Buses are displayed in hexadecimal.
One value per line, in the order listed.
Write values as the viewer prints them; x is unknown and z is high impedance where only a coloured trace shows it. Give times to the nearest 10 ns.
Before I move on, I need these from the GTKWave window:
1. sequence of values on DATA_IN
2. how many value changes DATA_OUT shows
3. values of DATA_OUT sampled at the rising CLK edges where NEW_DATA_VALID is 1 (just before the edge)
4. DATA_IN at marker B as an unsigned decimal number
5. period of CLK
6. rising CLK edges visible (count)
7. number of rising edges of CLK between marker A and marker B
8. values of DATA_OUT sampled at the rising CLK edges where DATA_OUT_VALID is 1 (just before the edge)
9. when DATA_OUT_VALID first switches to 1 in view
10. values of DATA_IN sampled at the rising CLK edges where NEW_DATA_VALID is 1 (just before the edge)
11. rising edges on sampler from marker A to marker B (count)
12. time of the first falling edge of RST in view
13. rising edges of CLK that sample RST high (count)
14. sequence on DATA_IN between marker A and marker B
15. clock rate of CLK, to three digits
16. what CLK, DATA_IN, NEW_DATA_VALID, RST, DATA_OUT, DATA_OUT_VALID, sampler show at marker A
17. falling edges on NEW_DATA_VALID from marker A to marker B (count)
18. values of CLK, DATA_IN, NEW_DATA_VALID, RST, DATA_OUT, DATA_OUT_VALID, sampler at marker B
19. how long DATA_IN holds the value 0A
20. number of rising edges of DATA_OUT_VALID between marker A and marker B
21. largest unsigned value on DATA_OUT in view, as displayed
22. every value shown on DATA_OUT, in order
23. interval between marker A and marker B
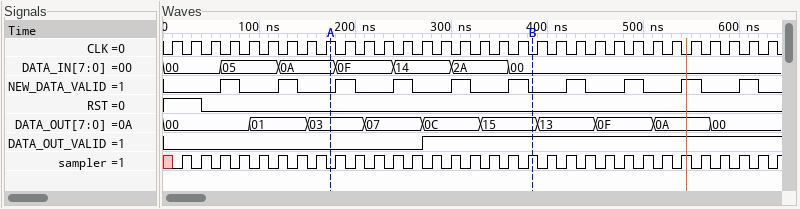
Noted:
00, 05, 0A, 0F, 14, 2A, 00
9
00, 01, 03, 07, 0C, 15, 13, 0F, 0A, 00
0
20 ns
32
10
0C, 0C, 0C, 15, 15, 15, 13, 13, 13, 0F, 0F, 0F, 0A, 0A, 0A, 00, 00, 00
270 ns
05, 0A, 0F, 14, 2A, 00, 00, 00, 00, 00
11
40 ns
2
0A, 0F, 14, 2A, 00
50.0 MHz
CLK=1, DATA_IN=0A, NEW_DATA_VALID=0, RST=0, DATA_OUT=03, DATA_OUT_VALID=0, sampler=0
4
CLK=0, DATA_IN=00, NEW_DATA_VALID=0, RST=0, DATA_OUT=15, DATA_OUT_VALID=1, sampler=1
60 ns
1
15
00, 01, 03, 07, 0C, 15, 13, 0F, 0A, 00
210 ns
